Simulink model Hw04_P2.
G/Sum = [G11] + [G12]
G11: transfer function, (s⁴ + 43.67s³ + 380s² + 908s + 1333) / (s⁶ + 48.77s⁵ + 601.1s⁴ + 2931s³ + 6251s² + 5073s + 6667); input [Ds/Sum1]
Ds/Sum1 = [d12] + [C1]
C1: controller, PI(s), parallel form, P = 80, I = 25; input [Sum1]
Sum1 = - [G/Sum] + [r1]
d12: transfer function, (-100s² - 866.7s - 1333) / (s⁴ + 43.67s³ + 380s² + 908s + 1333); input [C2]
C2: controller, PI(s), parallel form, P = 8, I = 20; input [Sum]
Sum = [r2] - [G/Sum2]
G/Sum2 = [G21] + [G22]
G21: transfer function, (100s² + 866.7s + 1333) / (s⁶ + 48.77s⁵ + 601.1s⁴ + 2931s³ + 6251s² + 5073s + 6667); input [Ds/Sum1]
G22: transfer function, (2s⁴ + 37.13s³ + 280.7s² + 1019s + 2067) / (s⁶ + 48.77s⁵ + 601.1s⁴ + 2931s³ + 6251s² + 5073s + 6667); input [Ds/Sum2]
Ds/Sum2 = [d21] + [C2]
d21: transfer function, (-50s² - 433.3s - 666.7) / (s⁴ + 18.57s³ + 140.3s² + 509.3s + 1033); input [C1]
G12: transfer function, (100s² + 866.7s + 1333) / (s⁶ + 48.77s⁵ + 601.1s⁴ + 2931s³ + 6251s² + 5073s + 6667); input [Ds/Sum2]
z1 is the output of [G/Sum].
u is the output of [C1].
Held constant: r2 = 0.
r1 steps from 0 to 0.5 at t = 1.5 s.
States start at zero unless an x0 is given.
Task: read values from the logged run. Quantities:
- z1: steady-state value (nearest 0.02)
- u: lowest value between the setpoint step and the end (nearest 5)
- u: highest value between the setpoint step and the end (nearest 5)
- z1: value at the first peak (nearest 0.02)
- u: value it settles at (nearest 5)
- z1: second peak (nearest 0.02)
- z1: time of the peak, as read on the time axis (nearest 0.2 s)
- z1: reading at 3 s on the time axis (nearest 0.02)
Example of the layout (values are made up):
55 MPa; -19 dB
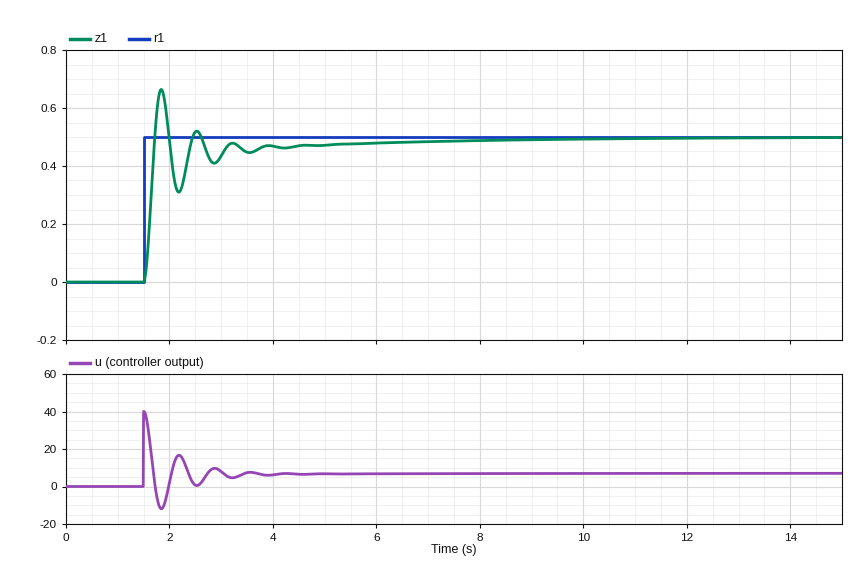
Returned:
0.50; -10; 40; 0.66; 5; 0.52; 1.8 s; 0.44
